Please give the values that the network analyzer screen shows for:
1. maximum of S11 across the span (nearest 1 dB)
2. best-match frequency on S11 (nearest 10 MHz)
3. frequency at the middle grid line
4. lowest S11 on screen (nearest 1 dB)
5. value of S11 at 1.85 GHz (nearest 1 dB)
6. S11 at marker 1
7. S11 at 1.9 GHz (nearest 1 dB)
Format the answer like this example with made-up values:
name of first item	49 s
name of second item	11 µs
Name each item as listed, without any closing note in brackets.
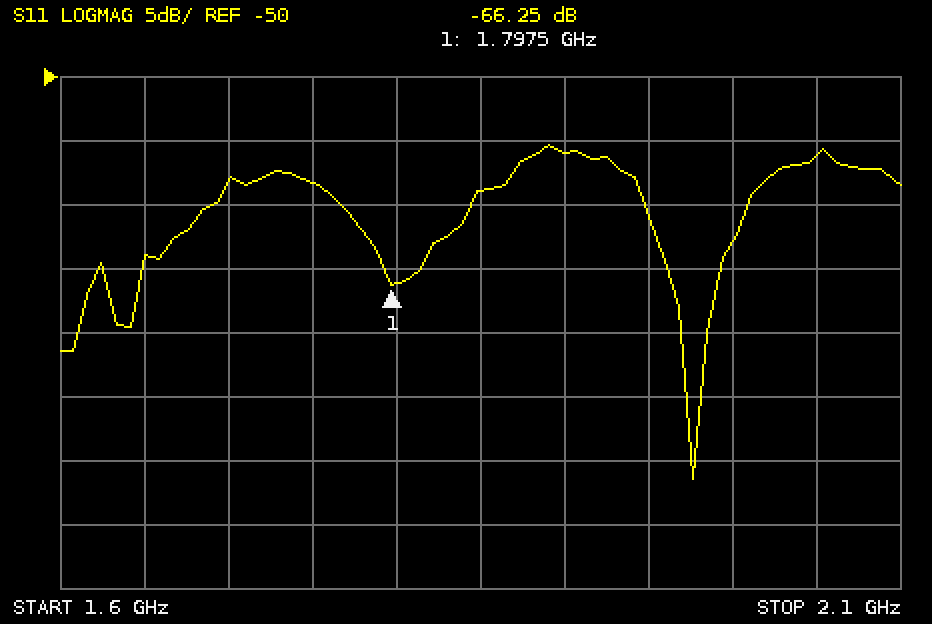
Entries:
maximum of S11 across the span	-55 dB
best-match frequency on S11	1.98 GHz
frequency at the middle grid line	1.85 GHz
lowest S11 on screen	-81 dB
value of S11 at 1.85 GHz	-59 dB
S11 at marker 1	-66.25 dB
S11 at 1.9 GHz	-56 dB
